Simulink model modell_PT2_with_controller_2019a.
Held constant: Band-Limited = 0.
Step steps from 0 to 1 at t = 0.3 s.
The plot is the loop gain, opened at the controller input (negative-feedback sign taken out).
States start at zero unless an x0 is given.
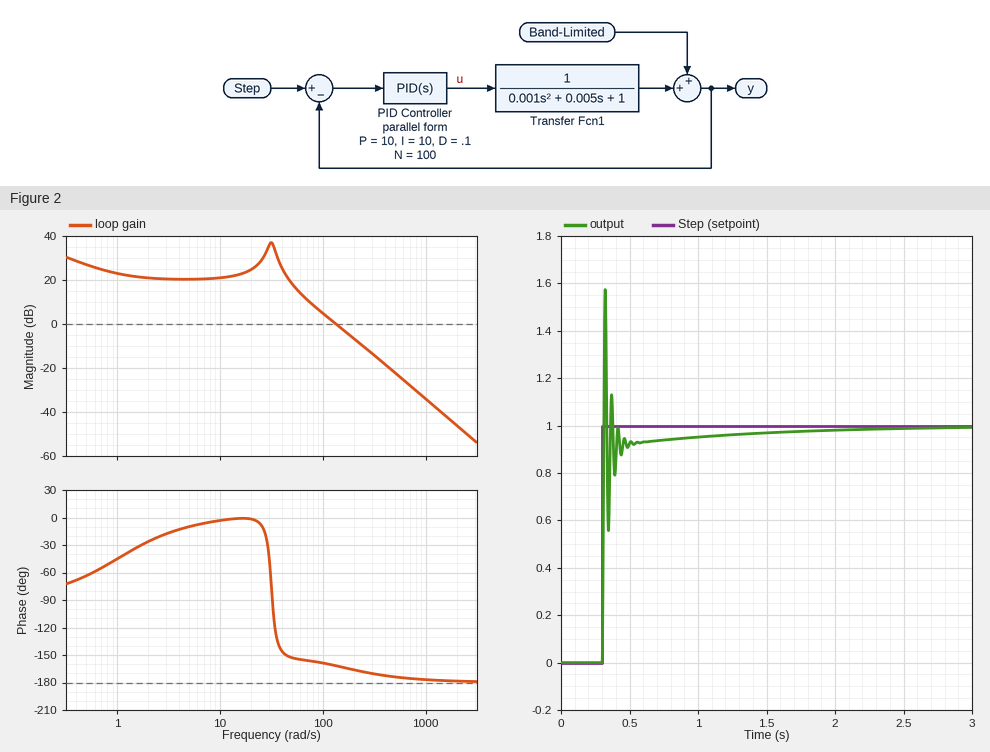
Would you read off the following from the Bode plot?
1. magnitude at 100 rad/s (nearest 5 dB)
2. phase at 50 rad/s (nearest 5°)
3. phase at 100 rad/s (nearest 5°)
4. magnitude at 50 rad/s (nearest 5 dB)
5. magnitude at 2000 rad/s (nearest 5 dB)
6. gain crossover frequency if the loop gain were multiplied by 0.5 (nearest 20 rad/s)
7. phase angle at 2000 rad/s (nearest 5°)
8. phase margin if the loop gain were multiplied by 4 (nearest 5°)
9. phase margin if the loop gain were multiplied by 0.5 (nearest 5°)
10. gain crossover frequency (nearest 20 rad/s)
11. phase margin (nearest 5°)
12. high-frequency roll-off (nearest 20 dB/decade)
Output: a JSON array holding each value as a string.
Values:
["5 dB", "-155°", "-160°", "20 dB", "-45 dB", "100 rad/s", "-180°", "10°", "20°", "140 rad/s", "20°", "-40 dB/decade"]
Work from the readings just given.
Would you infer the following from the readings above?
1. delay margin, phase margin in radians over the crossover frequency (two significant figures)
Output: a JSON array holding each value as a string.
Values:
["0.0025 s"]
